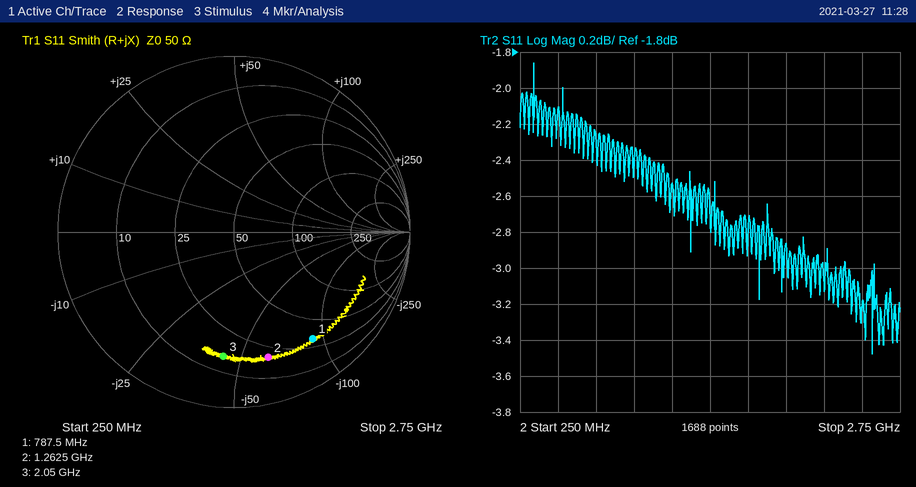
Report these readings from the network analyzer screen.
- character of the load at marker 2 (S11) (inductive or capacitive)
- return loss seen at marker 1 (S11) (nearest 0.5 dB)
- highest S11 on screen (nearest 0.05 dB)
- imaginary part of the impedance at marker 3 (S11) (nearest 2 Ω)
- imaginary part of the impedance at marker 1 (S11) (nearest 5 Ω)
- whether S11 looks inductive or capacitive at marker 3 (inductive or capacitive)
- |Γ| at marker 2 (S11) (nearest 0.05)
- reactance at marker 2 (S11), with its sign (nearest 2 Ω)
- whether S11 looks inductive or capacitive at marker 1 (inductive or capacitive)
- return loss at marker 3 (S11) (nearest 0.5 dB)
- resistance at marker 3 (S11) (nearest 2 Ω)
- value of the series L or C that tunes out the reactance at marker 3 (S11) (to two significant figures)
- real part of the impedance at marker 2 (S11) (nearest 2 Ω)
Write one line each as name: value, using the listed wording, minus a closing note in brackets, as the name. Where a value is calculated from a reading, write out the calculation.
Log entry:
character of the load at marker 2 (S11): capacitive
return loss seen at marker 1 (S11): 2.5 dB
highest S11 on screen: -1.85 dB
imaginary part of the impedance at marker 3 (S11): -44 Ω
imaginary part of the impedance at marker 1 (S11): -90 Ω
whether S11 looks inductive or capacitive at marker 3: capacitive
|Γ| at marker 2 (S11): 0.75
reactance at marker 2 (S11), with its sign: -62 Ω
whether S11 looks inductive or capacitive at marker 1: capacitive
return loss at marker 3 (S11): 3.0 dB
resistance at marker 3 (S11): 16 Ω
value of the series L or C that tunes out the reactance at marker 3 (S11): L = 44 Ω/(2π × 2.05 GHz) ≈ 3.4 nH
real part of the impedance at marker 2 (S11): 20 Ω
